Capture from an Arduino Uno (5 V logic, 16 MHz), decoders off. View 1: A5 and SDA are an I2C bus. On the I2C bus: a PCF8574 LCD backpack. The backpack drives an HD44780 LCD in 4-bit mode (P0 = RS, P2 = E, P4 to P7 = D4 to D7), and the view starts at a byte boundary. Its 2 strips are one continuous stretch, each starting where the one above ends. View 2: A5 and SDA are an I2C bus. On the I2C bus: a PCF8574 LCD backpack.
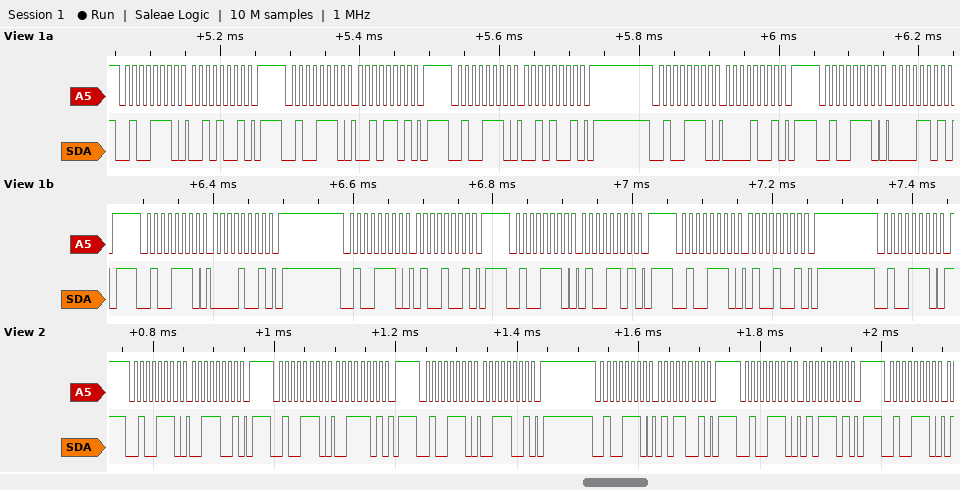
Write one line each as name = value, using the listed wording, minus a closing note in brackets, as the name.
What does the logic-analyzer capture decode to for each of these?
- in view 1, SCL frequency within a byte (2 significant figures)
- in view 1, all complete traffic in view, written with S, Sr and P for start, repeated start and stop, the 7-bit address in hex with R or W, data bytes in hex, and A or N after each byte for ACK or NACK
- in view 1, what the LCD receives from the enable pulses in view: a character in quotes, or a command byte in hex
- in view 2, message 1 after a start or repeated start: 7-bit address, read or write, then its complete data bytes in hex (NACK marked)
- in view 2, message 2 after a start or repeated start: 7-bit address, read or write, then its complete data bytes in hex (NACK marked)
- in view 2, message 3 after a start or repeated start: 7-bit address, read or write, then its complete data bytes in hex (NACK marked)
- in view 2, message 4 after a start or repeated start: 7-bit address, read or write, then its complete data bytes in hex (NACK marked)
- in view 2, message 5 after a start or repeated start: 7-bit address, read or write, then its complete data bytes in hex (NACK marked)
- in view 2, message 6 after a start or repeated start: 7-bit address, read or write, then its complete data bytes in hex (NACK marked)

in view 1, SCL frequency within a byte = 100 kHz
in view 1, all complete traffic in view, written with S, Sr and P for start, repeated start and stop, the 7-bit address in hex with R or W, data bytes in hex, and A or N after each byte for ACK or NACK = S 27W A 29 A P S 27W A 2D A P S 27W A 29 A P S 27W A 09 A P S 27W A 0D A P S 27W A 09 A P S 27W A 49 A P S 27W A 4D A P S 27W A 49 A P S 27W A
in view 1, what the LCD receives from the enable pulses in view: a character in quotes, or a command byte in hex = ' '
in view 2, message 1 after a start or repeated start: 7-bit address, read or write, then its complete data bytes in hex = 0x27 write: 39
in view 2, message 2 after a start or repeated start: 7-bit address, read or write, then its complete data bytes in hex = 0x27 write: 3D
in view 2, message 3 after a start or repeated start: 7-bit address, read or write, then its complete data bytes in hex = 0x27 write: 39
in view 2, message 4 after a start or repeated start: 7-bit address, read or write, then its complete data bytes in hex = 0x27 write: 59
in view 2, message 5 after a start or repeated start: 7-bit address, read or write, then its complete data bytes in hex = 0x27 write: 5D
in view 2, message 6 after a start or repeated start: 7-bit address, read or write, then its complete data bytes in hex = 0x27 write
